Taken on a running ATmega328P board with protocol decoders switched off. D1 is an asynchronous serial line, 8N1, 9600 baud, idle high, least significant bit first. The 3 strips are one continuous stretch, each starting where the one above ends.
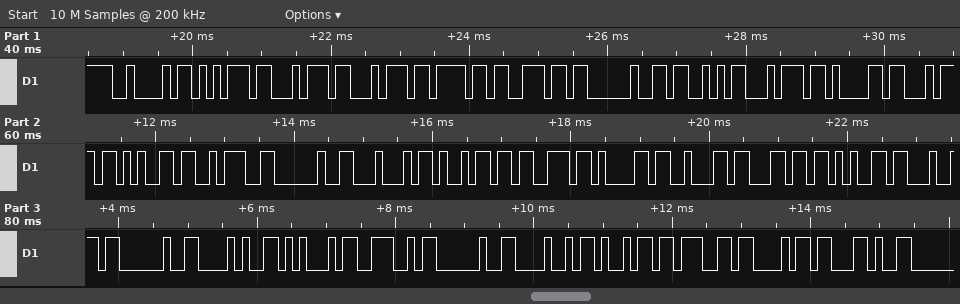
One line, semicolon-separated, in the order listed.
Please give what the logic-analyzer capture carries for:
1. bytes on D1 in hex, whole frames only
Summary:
42 75 74 74 6F 6E 20 53 74 61 74 65 3A 20 44 69 73 61 62 6C 65 64 20 28 45 4E 20 48 69 67 68 2C
